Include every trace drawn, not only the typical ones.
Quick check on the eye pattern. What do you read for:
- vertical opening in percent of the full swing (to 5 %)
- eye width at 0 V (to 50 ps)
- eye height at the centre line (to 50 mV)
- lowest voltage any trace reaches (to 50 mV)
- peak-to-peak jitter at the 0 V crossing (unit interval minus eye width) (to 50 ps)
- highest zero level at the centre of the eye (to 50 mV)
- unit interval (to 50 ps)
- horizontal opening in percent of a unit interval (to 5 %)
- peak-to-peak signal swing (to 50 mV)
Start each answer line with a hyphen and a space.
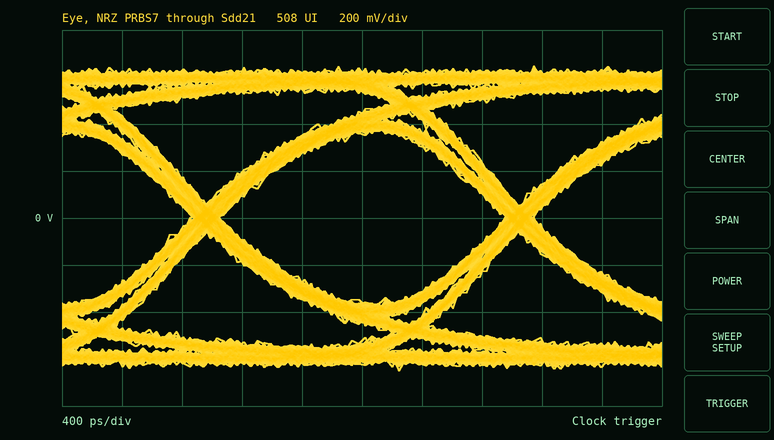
- 55 %
- 1.90 ns
- 700 mV
- -650 mV
- 200 ps
- -350 mV
- 2.10 ns
- 90 %
- 1.30 V
